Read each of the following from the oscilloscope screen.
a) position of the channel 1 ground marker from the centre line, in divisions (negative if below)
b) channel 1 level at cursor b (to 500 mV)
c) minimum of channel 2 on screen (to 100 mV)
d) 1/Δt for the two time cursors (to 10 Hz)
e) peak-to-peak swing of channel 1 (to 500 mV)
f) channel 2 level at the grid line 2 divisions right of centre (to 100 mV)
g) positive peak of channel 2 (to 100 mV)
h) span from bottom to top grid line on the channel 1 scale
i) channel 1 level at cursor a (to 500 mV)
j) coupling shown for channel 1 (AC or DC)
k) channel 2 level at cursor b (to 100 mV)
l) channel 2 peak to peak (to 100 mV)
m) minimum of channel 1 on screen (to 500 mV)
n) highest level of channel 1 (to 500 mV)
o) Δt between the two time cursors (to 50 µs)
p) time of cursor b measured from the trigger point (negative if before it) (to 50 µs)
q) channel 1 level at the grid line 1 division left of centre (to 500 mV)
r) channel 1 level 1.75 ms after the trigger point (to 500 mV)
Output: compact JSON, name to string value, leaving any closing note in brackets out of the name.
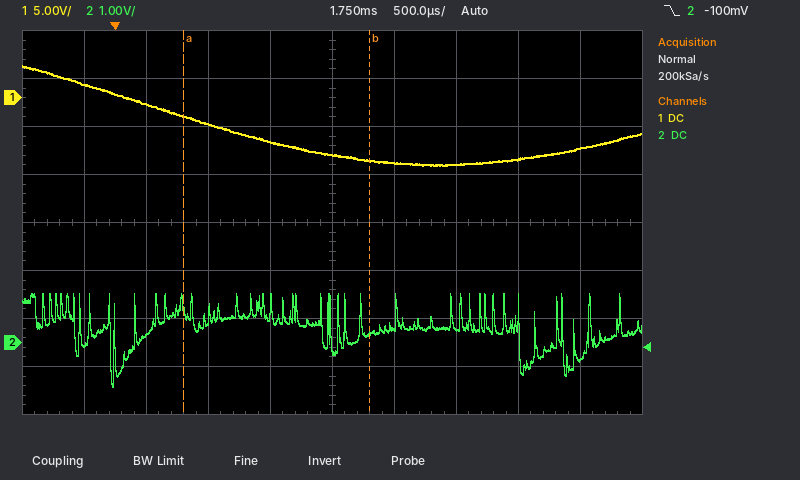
{"position of the channel 1 ground marker from the centre line, in divisions": "+2.6 div", "channel 1 level at cursor b": "-6.5 V", "minimum of channel 2 on screen": "-900 mV", "1/Δt for the two time cursors": "670 Hz", "peak-to-peak swing of channel 1": "10.5 V", "channel 2 level at the grid line 2 divisions right of centre": "300 mV", "positive peak of channel 2": "1.0 V", "span from bottom to top grid line on the channel 1 scale": "40 V", "channel 1 level at cursor a": "-2.0 V", "coupling shown for channel 1": "DC", "channel 2 level at cursor b": "200 mV", "channel 2 peak to peak": "1.9 V", "minimum of channel 1 on screen": "-7.0 V", "highest level of channel 1": "3.5 V", "Δt between the two time cursors": "1.50 ms", "time of cursor b measured from the trigger point (negative if before it)": "+2.05 ms", "channel 1 level at the grid line 1 division left of centre": "-4.5 V", "channel 1 level 1.75 ms after the trigger point": "-6.0 V"}
